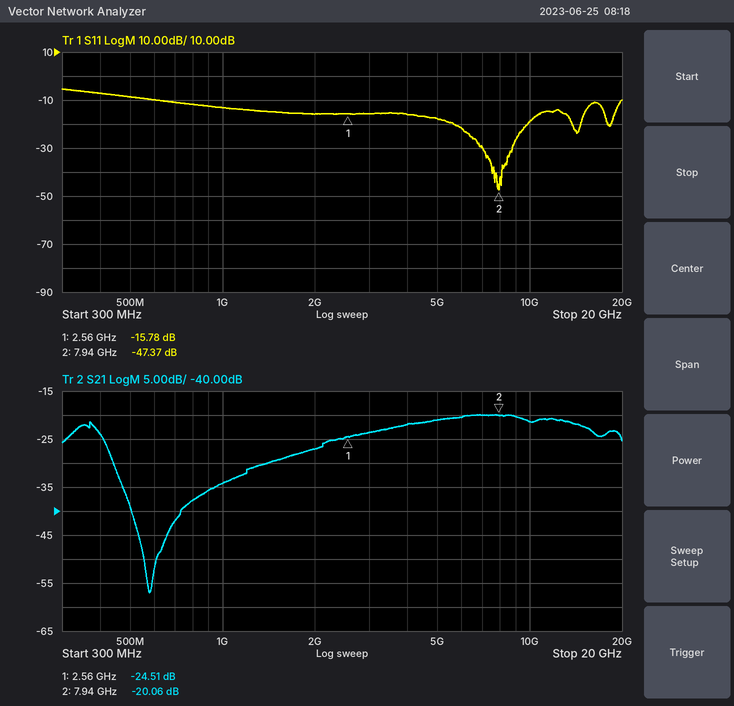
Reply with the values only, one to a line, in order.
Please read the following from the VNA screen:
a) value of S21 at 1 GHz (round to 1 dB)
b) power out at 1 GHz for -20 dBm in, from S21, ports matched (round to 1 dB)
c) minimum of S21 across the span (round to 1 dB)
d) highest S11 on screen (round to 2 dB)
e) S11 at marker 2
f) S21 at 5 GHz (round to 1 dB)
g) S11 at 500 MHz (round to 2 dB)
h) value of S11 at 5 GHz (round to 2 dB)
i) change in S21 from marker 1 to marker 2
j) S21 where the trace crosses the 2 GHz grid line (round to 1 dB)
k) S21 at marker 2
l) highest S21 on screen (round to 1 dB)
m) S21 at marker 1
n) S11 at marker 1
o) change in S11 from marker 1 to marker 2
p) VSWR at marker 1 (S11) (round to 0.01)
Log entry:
-34 dB
-54 dBm
-57 dB
-6 dB
-47.37 dB
-21 dB
-8 dB
-18 dB
4.45 dB
-27 dB
-20.06 dB
-20 dB
-24.51 dB
-15.78 dB
-31.59 dB
1.39
